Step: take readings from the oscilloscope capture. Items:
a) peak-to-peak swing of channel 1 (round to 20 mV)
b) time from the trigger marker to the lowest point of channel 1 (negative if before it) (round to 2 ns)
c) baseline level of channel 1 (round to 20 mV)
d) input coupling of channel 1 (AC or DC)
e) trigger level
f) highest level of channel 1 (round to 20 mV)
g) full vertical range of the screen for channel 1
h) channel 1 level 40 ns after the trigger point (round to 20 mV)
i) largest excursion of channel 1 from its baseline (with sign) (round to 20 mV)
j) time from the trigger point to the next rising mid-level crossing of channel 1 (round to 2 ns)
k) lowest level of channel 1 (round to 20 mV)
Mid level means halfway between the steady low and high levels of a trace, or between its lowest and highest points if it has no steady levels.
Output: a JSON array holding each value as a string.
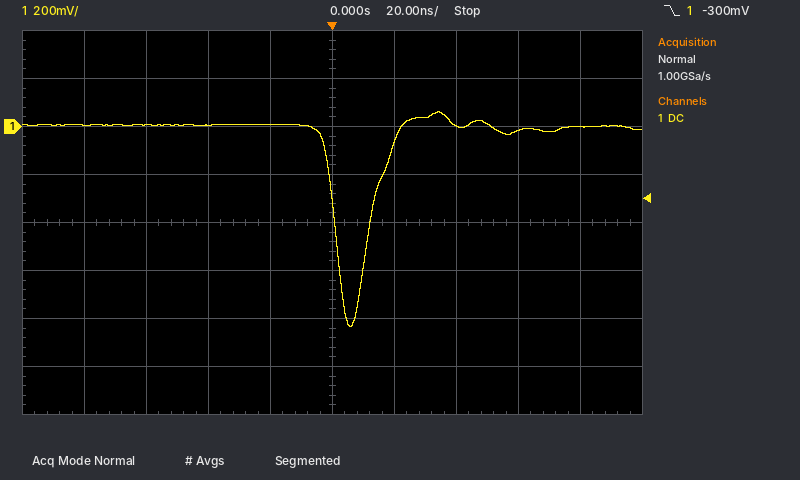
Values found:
["900 mV", "+6 ns", "0 mV", "DC", "-300 mV", "60 mV", "1.6 V", "0 mV", "-840 mV", "12 ns", "-840 mV"]
